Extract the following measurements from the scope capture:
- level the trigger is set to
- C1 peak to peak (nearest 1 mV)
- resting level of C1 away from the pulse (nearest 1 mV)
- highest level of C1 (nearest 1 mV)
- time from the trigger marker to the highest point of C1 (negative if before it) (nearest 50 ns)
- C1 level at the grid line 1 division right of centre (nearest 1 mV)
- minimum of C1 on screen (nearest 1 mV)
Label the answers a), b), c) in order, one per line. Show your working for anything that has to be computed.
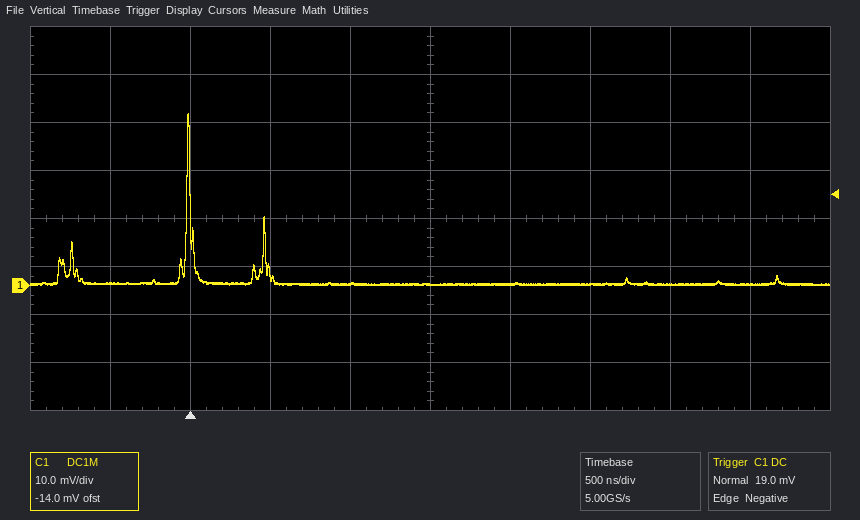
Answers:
a) 19.0 mV
b) 36 mV − (0 mV) = 36 mV
c) 0 mV
d) 36 mV
e) 0 ns
f) 0 mV
g) 0 mV
